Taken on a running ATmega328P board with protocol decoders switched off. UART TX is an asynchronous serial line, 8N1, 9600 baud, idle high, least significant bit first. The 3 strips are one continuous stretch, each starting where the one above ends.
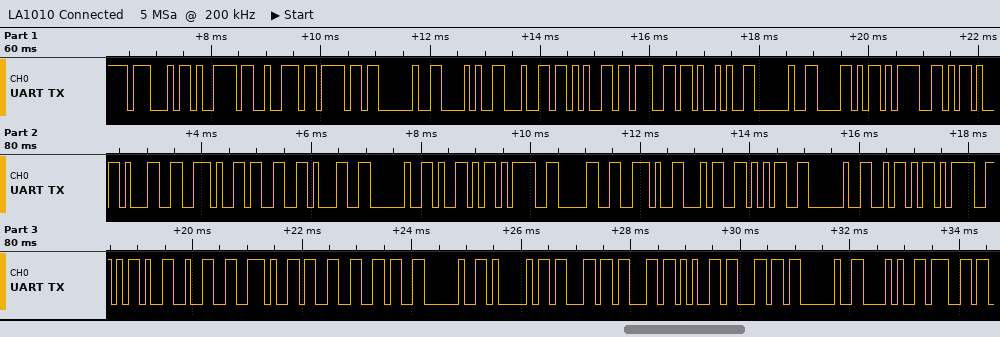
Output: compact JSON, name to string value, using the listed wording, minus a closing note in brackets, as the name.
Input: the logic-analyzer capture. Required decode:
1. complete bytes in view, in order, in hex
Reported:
{"complete bytes in view, in order, in hex": "47 79 72 6F 20 28 64 65 67 29 20 58 3D 2D 31 2E 33 31 20 59 3D 30 2E 34 35 20 5A 3D 2D 32 2E 33 36 20 41 63 63 65 6C 20 28 67"}
